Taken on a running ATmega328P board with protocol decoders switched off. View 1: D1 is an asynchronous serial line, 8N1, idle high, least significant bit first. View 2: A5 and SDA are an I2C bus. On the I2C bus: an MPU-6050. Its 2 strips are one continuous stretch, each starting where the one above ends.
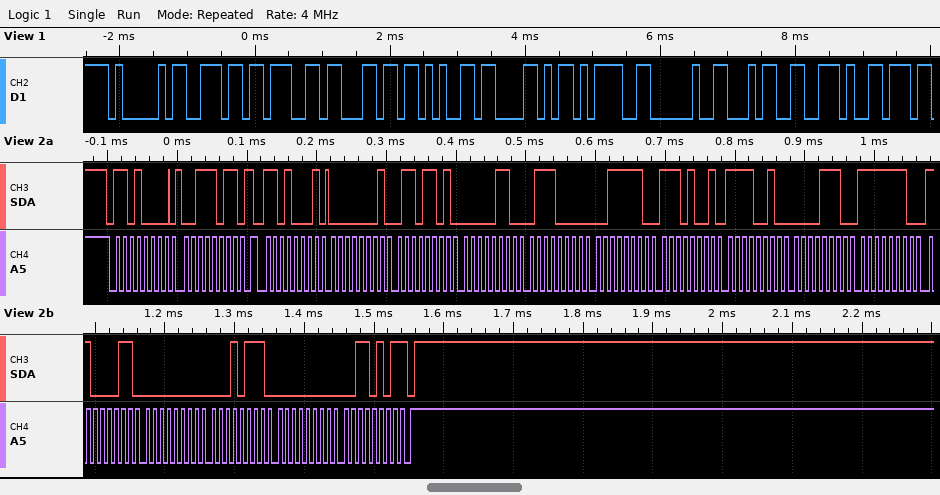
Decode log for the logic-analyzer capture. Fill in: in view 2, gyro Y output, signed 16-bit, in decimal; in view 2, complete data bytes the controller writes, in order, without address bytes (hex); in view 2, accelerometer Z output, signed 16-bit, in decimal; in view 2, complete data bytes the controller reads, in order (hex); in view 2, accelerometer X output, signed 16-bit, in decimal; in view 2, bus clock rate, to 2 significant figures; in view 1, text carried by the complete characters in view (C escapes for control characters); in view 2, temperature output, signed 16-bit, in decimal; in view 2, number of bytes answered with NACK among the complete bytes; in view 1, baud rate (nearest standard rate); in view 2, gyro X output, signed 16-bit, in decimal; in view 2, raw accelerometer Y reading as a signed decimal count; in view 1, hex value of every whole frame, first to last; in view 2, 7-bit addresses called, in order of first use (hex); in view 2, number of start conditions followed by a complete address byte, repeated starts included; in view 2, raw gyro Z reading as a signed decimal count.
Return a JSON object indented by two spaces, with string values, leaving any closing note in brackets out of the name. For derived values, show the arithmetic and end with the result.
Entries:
{
  "in view 2, gyro Y output, signed 16-bit, in decimal": "0x0017 = 23",
  "in view 2, complete data bytes the controller writes, in order, without address bytes": "3B",
  "in view 2, accelerometer Z output, signed 16-bit, in decimal": "0x3EE9 = 16105",
  "in view 2, complete data bytes the controller reads, in order": "01 6D 06 70 3E E9 F2 0E FE C3 00 17 00 35",
  "in view 2, accelerometer X output, signed 16-bit, in decimal": "0x016D = 365",
  "in view 2, bus clock rate, to 2 significant figures": "100 kHz",
  "in view 1, text carried by the complete characters in view": "\"AngleX= 4.\"",
  "in view 2, temperature output, signed 16-bit, in decimal": "0xF20E = -3570",
  "in view 2, number of bytes answered with NACK among the complete bytes": "1",
  "in view 1, baud rate": "9600 baud",
  "in view 2, gyro X output, signed 16-bit, in decimal": "0xFEC3 = -317",
  "in view 2, raw accelerometer Y reading as a signed decimal count": "0x0670 = 1648",
  "in view 1, hex value of every whole frame, first to last": "41 6E 67 6C 65 58 3D 20 34 2E",
  "in view 2, 7-bit addresses called, in order of first use": "0x68",
  "in view 2, number of start conditions followed by a complete address byte, repeated starts included": "2",
  "in view 2, raw gyro Z reading as a signed decimal count": "0x0035 = 53"
}
